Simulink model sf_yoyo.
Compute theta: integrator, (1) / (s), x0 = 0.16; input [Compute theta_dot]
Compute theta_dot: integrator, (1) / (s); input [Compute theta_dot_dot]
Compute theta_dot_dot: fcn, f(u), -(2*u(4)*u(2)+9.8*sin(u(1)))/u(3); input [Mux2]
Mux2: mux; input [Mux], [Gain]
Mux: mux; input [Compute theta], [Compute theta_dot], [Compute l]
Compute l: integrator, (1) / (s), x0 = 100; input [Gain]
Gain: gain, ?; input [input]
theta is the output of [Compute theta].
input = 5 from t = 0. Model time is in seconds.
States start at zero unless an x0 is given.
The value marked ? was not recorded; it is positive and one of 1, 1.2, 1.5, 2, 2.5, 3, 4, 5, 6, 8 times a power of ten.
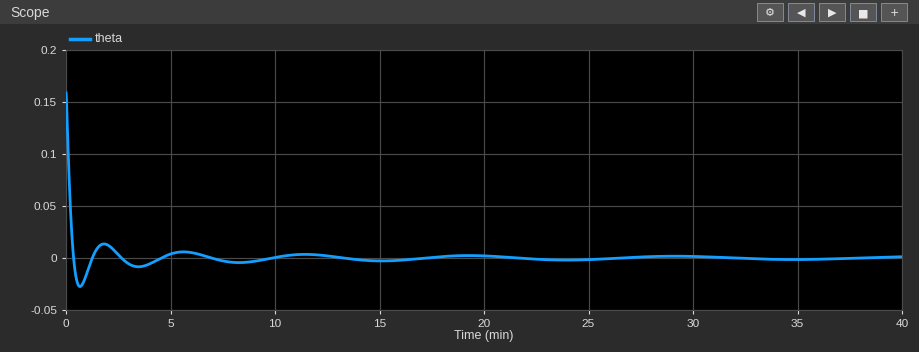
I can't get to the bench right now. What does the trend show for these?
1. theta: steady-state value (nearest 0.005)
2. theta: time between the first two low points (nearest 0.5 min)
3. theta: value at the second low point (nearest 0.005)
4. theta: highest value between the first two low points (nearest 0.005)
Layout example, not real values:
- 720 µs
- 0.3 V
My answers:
- 0.000
- 3.0 min
- -0.010
- 0.015
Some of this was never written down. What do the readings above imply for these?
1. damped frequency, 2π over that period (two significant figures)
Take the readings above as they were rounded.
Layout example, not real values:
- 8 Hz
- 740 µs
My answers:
- 2.1 rad/min
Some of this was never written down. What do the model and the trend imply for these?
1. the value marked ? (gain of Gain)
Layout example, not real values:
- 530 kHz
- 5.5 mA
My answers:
- 12
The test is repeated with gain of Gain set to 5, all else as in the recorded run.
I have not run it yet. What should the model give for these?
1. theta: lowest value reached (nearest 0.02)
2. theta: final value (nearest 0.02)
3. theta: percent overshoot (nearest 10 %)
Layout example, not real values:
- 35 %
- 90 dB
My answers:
- -0.04
- 0.00
- 30 %
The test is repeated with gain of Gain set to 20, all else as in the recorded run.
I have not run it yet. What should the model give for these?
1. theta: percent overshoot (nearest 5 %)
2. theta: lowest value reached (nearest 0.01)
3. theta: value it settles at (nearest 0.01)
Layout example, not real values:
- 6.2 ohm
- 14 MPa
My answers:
- 15 %
- -0.02
- 0.00
